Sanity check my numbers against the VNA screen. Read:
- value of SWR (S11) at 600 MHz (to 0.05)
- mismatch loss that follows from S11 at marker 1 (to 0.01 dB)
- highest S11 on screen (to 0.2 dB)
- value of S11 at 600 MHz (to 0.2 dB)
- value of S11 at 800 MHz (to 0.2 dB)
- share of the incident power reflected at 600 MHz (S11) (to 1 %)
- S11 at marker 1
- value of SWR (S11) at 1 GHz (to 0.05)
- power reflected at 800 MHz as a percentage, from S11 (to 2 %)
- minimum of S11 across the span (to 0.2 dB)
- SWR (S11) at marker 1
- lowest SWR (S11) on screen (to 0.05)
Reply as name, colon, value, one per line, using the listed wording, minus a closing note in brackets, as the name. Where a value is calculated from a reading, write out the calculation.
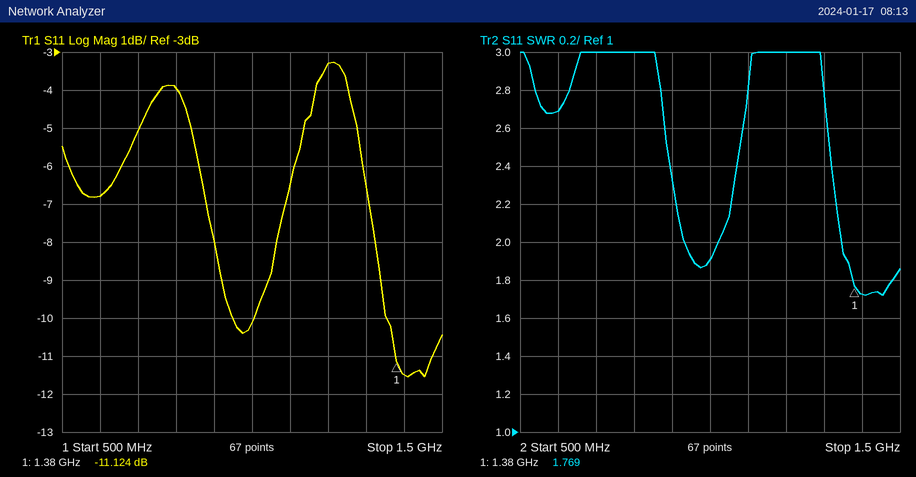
value of SWR (S11) at 600 MHz: 2.70
mismatch loss that follows from S11 at marker 1: −10 log10(1 − 10^(-11.124/10)) ≈ 0.35 dB
highest S11 on screen: -3.2 dB
value of S11 at 600 MHz: -6.8 dB
value of S11 at 800 MHz: -4.0 dB
share of the incident power reflected at 600 MHz (S11): 10^(-6.8/10) ≈ 21 %
S11 at marker 1: -11.124 dB
value of SWR (S11) at 1 GHz: 1.90
power reflected at 800 MHz as a percentage, from S11: 10^(-4/10) ≈ 40 %
minimum of S11 across the span: -11.6 dB
SWR (S11) at marker 1: 1.769
lowest SWR (S11) on screen: 1.70
